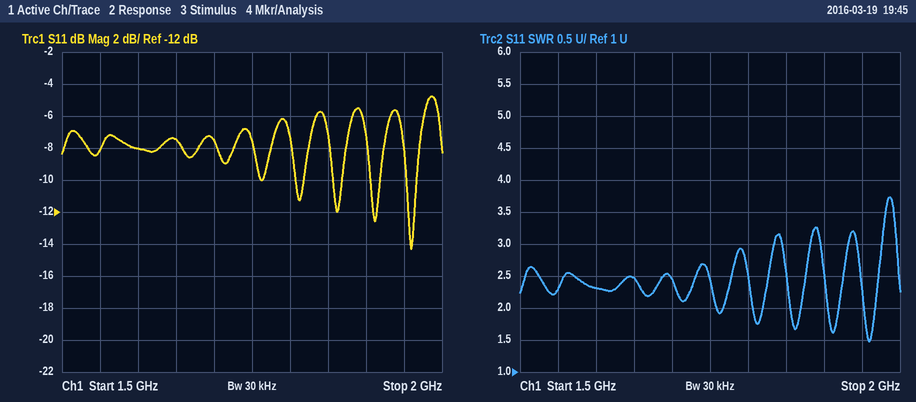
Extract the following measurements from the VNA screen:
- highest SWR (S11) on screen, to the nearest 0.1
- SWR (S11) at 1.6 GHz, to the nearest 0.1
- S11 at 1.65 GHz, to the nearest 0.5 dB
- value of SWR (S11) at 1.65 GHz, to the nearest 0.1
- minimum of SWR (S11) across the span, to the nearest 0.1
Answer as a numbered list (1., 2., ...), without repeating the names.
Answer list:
1. 3.7
2. 2.3
3. -7.5 dB
4. 2.5
5. 1.5
